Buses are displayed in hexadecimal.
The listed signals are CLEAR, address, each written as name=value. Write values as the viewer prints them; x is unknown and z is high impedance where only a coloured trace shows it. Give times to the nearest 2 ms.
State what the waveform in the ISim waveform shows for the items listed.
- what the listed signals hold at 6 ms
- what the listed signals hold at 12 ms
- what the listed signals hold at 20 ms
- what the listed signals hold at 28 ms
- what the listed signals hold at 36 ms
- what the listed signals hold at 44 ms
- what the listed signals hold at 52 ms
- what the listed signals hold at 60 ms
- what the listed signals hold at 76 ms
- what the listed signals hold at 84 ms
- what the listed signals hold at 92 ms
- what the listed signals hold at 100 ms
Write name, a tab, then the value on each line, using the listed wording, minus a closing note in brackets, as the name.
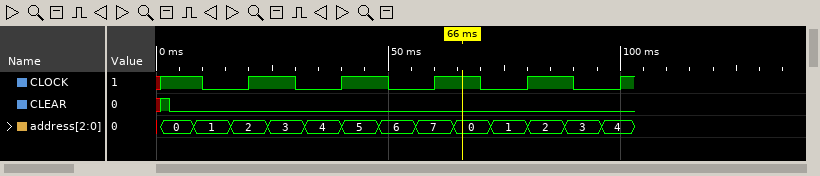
what the listed signals hold at 6 ms	CLEAR=0, address=0
what the listed signals hold at 12 ms	CLEAR=0, address=1
what the listed signals hold at 20 ms	CLEAR=0, address=2
what the listed signals hold at 28 ms	CLEAR=0, address=3
what the listed signals hold at 36 ms	CLEAR=0, address=4
what the listed signals hold at 44 ms	CLEAR=0, address=5
what the listed signals hold at 52 ms	CLEAR=0, address=6
what the listed signals hold at 60 ms	CLEAR=0, address=7
what the listed signals hold at 76 ms	CLEAR=0, address=1
what the listed signals hold at 84 ms	CLEAR=0, address=2
what the listed signals hold at 92 ms	CLEAR=0, address=3
what the listed signals hold at 100 ms	CLEAR=0, address=4
